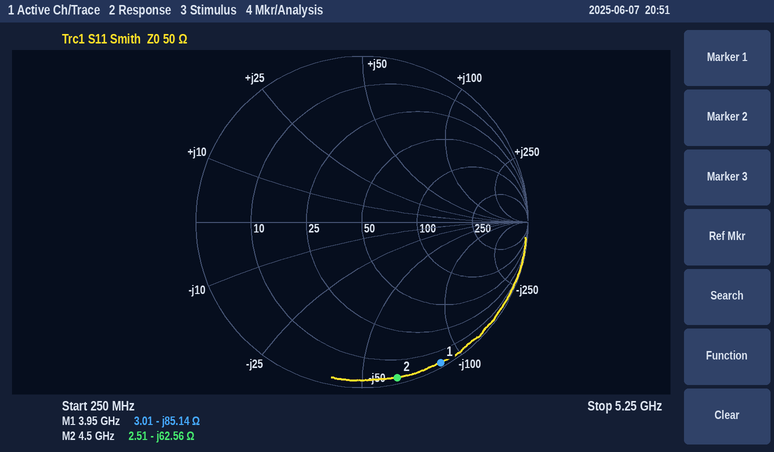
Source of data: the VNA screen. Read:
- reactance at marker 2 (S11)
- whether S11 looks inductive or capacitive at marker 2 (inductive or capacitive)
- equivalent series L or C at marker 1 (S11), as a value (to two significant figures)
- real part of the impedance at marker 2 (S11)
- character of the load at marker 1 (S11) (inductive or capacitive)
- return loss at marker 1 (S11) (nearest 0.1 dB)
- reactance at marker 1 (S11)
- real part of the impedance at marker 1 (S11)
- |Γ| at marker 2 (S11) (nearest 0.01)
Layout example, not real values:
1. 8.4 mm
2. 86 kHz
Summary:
1. -62.56 Ω
2. capacitive
3. 470 fF
4. 2.51 Ω
5. capacitive
6. 0.3 dB
7. -85.14 Ω
8. 3.01 Ω
9. 0.96
